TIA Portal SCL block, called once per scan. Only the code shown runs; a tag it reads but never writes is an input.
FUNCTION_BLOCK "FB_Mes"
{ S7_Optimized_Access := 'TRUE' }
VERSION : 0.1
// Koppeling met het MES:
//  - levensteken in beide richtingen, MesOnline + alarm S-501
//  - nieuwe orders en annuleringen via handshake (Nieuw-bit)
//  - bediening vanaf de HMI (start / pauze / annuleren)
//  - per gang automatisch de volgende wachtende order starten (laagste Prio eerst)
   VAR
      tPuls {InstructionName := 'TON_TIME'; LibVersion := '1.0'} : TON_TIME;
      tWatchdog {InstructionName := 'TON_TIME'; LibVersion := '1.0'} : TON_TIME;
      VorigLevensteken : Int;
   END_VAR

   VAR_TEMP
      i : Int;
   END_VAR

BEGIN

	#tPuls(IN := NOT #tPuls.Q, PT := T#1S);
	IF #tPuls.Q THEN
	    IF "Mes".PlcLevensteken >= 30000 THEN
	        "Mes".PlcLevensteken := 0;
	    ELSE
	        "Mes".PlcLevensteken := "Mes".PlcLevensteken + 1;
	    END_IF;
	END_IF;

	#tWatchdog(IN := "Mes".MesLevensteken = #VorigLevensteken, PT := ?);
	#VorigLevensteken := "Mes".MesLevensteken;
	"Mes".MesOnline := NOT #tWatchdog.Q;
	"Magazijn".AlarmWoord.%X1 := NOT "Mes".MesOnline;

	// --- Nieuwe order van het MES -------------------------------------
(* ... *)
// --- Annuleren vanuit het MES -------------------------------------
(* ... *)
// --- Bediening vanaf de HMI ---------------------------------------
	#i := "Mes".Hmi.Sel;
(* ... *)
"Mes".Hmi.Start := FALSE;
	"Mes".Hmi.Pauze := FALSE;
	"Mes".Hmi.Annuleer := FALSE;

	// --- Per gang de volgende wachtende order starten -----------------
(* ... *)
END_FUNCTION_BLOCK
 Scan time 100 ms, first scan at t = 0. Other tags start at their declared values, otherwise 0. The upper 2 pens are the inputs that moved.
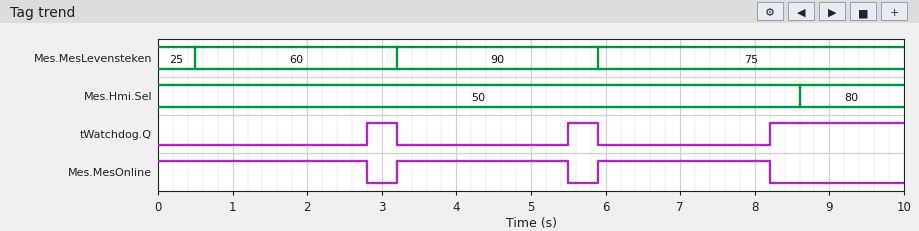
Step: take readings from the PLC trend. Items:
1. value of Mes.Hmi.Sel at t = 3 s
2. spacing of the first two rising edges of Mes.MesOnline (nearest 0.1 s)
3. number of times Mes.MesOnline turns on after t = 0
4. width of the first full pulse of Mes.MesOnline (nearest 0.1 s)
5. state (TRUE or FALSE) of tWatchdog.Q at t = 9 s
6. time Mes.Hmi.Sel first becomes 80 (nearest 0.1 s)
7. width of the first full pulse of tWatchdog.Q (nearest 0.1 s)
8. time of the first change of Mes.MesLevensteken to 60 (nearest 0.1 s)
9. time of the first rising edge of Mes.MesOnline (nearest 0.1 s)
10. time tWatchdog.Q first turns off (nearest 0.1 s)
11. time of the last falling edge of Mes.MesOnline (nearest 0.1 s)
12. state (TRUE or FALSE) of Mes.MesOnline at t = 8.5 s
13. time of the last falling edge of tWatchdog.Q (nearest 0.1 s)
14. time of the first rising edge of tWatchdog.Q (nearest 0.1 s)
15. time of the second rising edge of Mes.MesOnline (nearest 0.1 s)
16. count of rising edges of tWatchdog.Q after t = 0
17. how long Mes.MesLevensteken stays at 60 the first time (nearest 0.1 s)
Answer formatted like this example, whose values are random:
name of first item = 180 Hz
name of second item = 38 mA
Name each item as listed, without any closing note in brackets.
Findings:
value of Mes.Hmi.Sel at t = 3 s = 50
spacing of the first two rising edges of Mes.MesOnline = 2.7 s
number of times Mes.MesOnline turns on after t = 0 = 2
width of the first full pulse of Mes.MesOnline = 2.3 s
state (TRUE or FALSE) of tWatchdog.Q at t = 9 s = TRUE
time Mes.Hmi.Sel first becomes 80 = 8.6 s
width of the first full pulse of tWatchdog.Q = 0.4 s
time of the first change of Mes.MesLevensteken to 60 = 0.5 s
time of the first rising edge of Mes.MesOnline = 3.2 s
time tWatchdog.Q first turns off = 3.2 s
time of the last falling edge of Mes.MesOnline = 8.2 s
state (TRUE or FALSE) of Mes.MesOnline at t = 8.5 s = FALSE
time of the last falling edge of tWatchdog.Q = 5.9 s
time of the first rising edge of tWatchdog.Q = 2.8 s
time of the second rising edge of Mes.MesOnline = 5.9 s
count of rising edges of tWatchdog.Q after t = 0 = 3
how long Mes.MesLevensteken stays at 60 the first time = 2.7 s
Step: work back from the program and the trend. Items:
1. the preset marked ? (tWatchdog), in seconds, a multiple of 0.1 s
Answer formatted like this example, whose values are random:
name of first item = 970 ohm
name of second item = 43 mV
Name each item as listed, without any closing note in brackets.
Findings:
the preset marked ? (tWatchdog), in seconds, a multiple of 0.1 s = 2.2 s
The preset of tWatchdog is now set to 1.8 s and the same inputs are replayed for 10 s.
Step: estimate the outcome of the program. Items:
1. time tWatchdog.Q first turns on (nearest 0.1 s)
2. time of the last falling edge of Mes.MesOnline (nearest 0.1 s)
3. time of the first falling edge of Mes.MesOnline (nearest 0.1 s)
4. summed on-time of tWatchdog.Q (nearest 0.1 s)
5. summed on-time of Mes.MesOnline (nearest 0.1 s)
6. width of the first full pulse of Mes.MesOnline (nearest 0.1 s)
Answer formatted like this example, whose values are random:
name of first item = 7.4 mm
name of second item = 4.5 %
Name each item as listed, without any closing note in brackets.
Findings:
time tWatchdog.Q first turns on = 2.4 s
time of the last falling edge of Mes.MesOnline = 7.8 s
time of the first falling edge of Mes.MesOnline = 2.4 s
summed on-time of tWatchdog.Q = 3.8 s
summed on-time of Mes.MesOnline = 6.2 s
width of the first full pulse of Mes.MesOnline = 1.9 s
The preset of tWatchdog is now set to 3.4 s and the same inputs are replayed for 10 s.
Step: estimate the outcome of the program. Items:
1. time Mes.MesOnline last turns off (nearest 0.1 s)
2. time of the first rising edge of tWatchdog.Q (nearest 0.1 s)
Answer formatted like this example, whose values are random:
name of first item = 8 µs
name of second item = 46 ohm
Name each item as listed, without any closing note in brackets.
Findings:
time Mes.MesOnline last turns off = 9.4 s
time of the first rising edge of tWatchdog.Q = 9.4 s
